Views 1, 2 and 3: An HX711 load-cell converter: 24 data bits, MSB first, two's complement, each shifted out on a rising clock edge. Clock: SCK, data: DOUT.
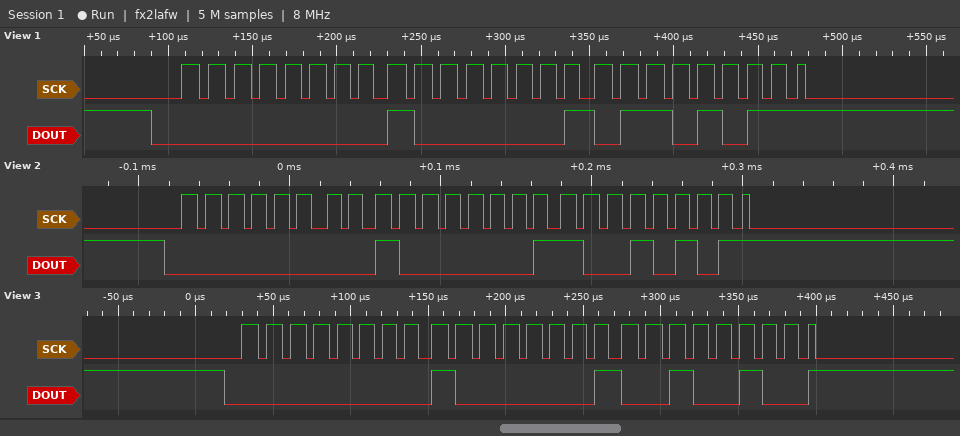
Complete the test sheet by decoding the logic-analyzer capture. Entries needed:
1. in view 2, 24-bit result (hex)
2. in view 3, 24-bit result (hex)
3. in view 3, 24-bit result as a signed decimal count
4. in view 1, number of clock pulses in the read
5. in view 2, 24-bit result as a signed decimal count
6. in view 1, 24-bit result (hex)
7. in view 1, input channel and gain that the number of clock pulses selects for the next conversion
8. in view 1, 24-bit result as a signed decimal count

0x008195
0x008124
33060
25
33173
0x00816B
channel A, gain 128
33131
